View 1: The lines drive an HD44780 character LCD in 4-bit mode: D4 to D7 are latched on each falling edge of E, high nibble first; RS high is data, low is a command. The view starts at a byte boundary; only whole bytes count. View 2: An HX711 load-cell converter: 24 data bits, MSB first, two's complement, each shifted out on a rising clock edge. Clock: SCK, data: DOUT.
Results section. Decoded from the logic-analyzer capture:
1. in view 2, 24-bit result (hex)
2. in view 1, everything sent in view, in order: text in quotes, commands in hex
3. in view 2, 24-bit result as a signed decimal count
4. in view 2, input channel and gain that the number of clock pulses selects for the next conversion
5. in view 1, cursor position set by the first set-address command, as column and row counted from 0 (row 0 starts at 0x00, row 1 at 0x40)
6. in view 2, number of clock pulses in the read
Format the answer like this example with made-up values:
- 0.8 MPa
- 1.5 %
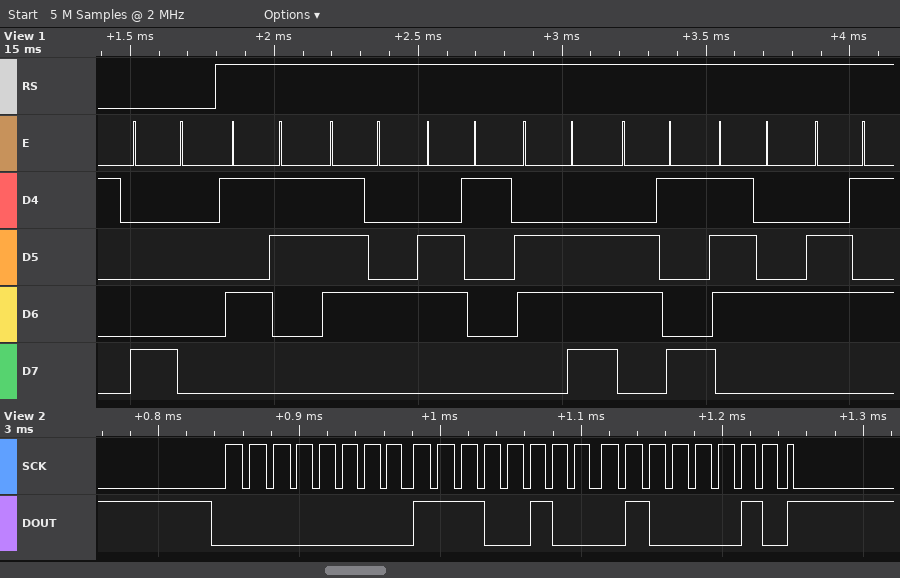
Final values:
- 0x00E442
- 0x80 "Stanite"
- 58434
- channel A, gain 128
- column 0, row 0
- 25
